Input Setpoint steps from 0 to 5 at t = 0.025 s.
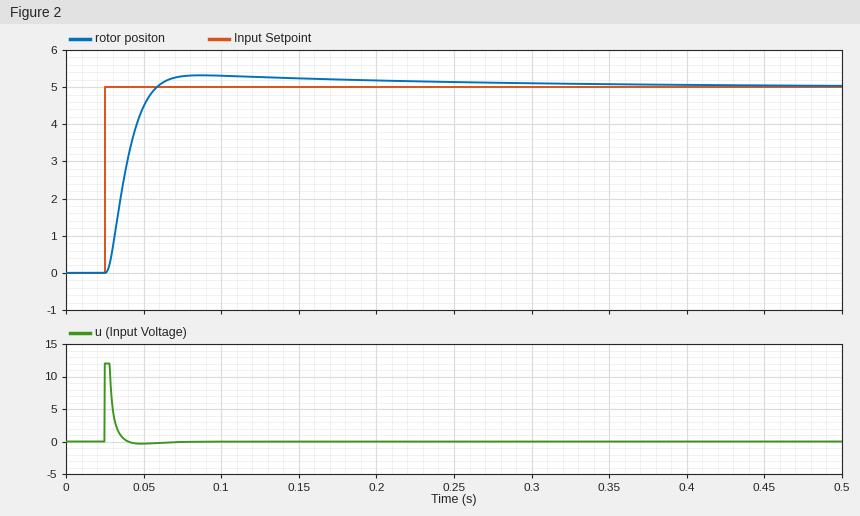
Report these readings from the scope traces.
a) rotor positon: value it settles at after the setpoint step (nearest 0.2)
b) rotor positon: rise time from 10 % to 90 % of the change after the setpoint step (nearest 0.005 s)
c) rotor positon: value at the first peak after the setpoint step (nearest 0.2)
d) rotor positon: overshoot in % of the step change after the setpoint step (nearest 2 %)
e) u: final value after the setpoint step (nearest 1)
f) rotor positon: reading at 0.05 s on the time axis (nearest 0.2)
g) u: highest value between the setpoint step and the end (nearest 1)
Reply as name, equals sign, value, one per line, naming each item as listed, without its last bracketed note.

rotor positon: value it settles at after the setpoint step = 5.0
rotor positon: rise time from 10 % to 90 % of the change after the setpoint step = 0.020 s
rotor positon: value at the first peak after the setpoint step = 5.4
rotor positon: overshoot in % of the step change after the setpoint step = 6 %
u: final value after the setpoint step = 0
rotor positon: reading at 0.05 s on the time axis = 4.4
u: highest value between the setpoint step and the end = 12
